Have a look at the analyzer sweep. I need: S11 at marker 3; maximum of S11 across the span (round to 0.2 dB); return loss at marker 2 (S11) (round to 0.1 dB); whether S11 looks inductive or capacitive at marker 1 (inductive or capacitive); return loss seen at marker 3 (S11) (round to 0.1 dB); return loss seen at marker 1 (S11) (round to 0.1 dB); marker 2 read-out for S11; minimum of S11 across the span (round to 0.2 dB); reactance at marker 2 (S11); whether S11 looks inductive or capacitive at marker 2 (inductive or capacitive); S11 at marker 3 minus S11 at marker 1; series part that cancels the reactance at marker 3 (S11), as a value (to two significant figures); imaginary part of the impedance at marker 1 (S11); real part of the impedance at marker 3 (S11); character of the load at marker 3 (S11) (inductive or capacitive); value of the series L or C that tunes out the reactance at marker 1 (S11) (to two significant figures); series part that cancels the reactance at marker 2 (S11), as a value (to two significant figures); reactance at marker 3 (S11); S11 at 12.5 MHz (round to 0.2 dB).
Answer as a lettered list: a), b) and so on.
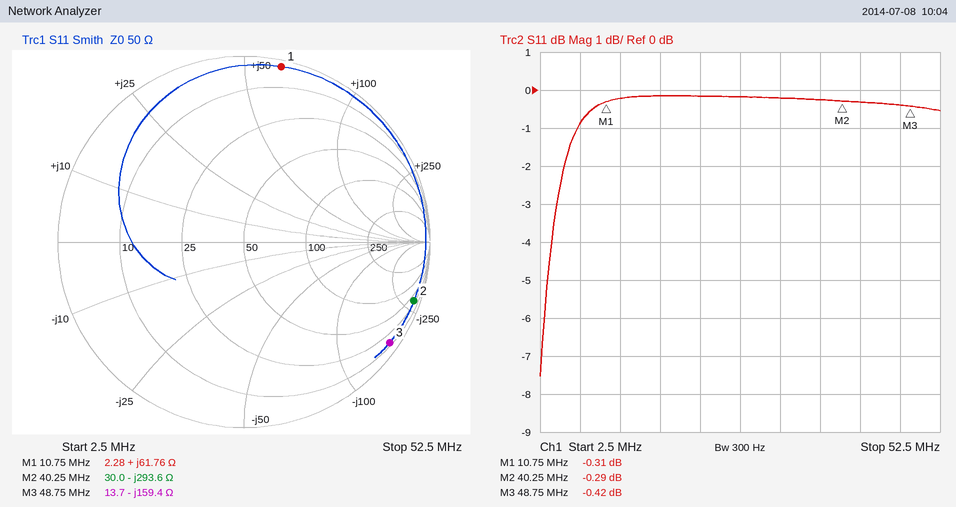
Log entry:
a) -0.42 dB
b) -0.2 dB
c) 0.3 dB
d) inductive
e) 0.4 dB
f) 0.3 dB
g) -0.29 dB
h) -7.6 dB
i) -293.6 Ω
j) capacitive
k) -0.11 dB
l) 520 nH
m) +61.76 Ω
n) 13.7 Ω
o) capacitive
p) 240 pF
q) 1.2 µH
r) -159.4 Ω
s) -0.2 dB
